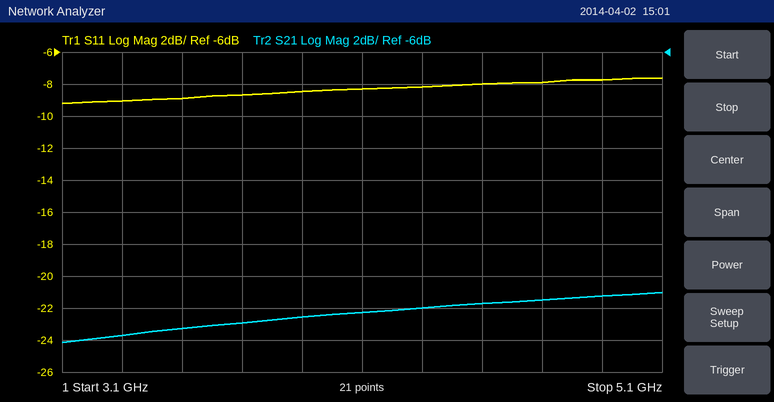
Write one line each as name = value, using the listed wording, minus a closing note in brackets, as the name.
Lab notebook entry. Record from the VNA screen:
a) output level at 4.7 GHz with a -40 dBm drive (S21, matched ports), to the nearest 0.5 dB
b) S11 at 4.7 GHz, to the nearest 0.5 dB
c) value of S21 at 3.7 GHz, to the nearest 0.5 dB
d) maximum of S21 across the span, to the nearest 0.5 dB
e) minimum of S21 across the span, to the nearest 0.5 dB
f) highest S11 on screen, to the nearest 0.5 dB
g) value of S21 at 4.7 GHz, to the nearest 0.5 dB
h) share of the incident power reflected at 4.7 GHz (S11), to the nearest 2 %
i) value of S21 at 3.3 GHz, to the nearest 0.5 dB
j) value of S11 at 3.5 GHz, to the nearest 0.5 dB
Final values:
output level at 4.7 GHz with a -40 dBm drive (S21, matched ports), to the nearest 0.5 dB = -61.5 dBm
S11 at 4.7 GHz, to the nearest 0.5 dB = -8.0 dB
value of S21 at 3.7 GHz, to the nearest 0.5 dB = -23.0 dB
maximum of S21 across the span, to the nearest 0.5 dB = -21.0 dB
minimum of S21 across the span, to the nearest 0.5 dB = -24.0 dB
highest S11 on screen, to the nearest 0.5 dB = -7.5 dB
value of S21 at 4.7 GHz, to the nearest 0.5 dB = -21.5 dB
share of the incident power reflected at 4.7 GHz (S11), to the nearest 2 % = 16 %
value of S21 at 3.3 GHz, to the nearest 0.5 dB = -23.5 dB
value of S11 at 3.5 GHz, to the nearest 0.5 dB = -9.0 dB
